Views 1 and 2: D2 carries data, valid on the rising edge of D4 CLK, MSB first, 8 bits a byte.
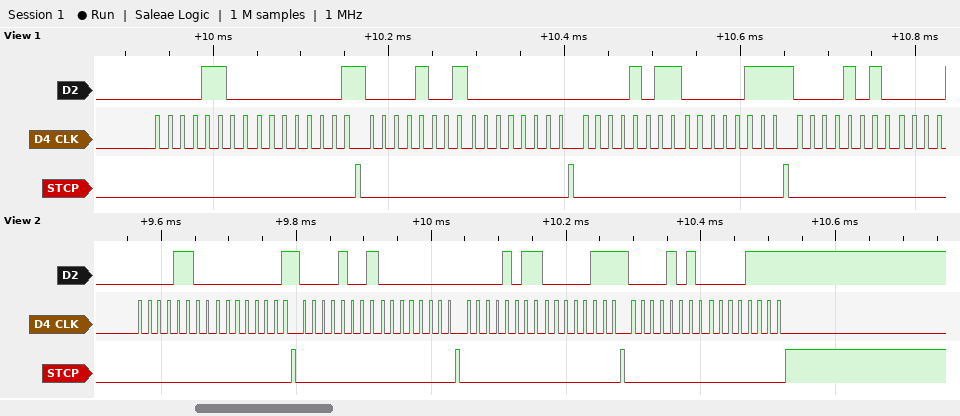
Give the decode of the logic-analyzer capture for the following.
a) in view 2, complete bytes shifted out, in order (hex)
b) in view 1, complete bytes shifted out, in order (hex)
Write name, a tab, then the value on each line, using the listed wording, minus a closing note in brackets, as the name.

in view 2, complete bytes shifted out, in order	0x0C 0x01 0x09 0x00 0x0B 0x07 0x0A 0x0F
in view 1, complete bytes shifted out, in order	0C 01 09 00 0B 07 0A
